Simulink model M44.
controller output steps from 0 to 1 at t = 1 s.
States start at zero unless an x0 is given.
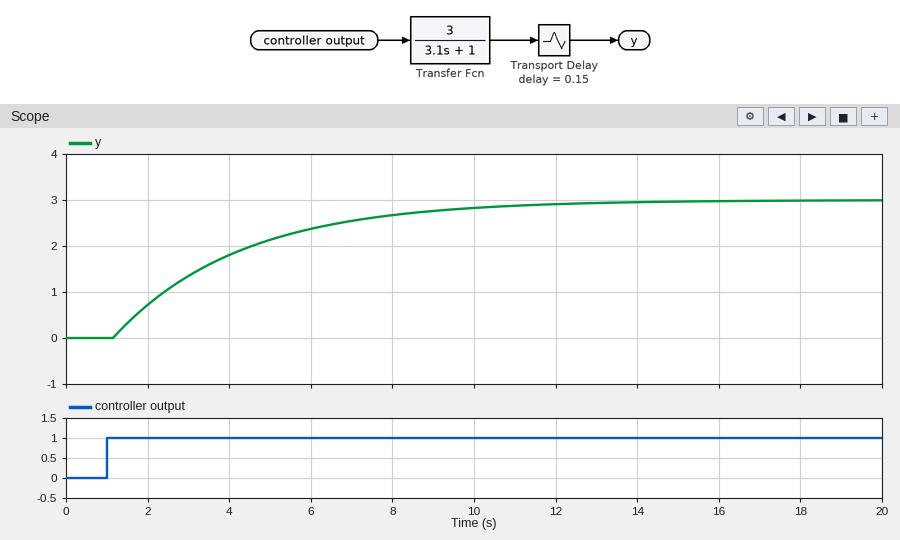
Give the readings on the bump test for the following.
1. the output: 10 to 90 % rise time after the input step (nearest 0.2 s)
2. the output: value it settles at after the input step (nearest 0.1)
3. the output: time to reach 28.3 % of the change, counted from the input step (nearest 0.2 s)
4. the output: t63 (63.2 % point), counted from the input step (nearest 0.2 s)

6.8 s
3.0
1.2 s
3.2 s
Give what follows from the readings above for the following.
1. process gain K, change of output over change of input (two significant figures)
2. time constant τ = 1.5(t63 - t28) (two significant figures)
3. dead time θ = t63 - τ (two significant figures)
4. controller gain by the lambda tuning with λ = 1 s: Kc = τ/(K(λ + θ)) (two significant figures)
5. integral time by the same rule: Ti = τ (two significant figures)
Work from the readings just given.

3.0
3.0 s
0.20 s
0.83
3.0 s
